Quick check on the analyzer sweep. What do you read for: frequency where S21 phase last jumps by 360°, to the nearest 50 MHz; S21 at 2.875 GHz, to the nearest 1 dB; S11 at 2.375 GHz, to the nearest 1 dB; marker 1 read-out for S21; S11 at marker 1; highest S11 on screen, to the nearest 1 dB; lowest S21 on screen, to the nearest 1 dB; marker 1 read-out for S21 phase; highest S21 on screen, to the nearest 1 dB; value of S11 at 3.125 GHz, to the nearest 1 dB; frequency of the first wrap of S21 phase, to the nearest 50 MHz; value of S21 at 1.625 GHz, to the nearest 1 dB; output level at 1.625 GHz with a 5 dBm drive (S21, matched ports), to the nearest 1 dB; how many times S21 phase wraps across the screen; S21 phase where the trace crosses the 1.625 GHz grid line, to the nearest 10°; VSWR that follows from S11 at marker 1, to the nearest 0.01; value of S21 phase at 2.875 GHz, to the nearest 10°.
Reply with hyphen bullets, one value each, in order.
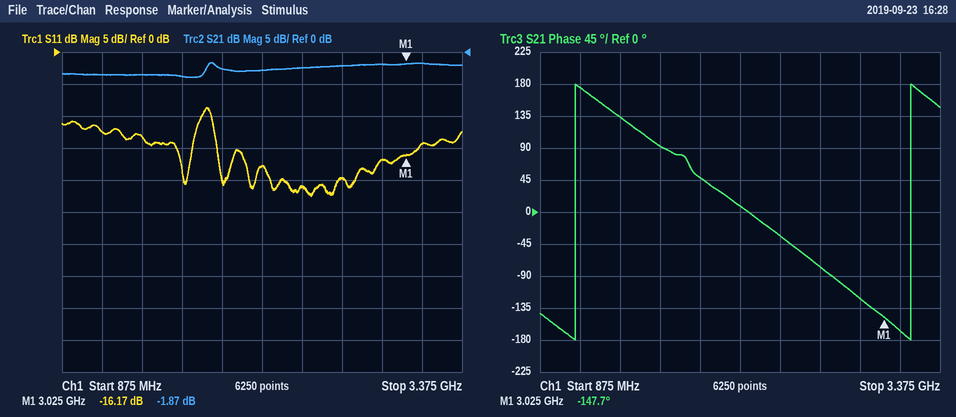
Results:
- 3.20 GHz
- -2 dB
- -21 dB
- -1.87 dB
- -16.17 dB
- -9 dB
- -4 dB
- -147.7°
- -2 dB
- -14 dB
- 1.10 GHz
- -4 dB
- 1 dBm
- 2
- 90°
- 1.37
- -120°
